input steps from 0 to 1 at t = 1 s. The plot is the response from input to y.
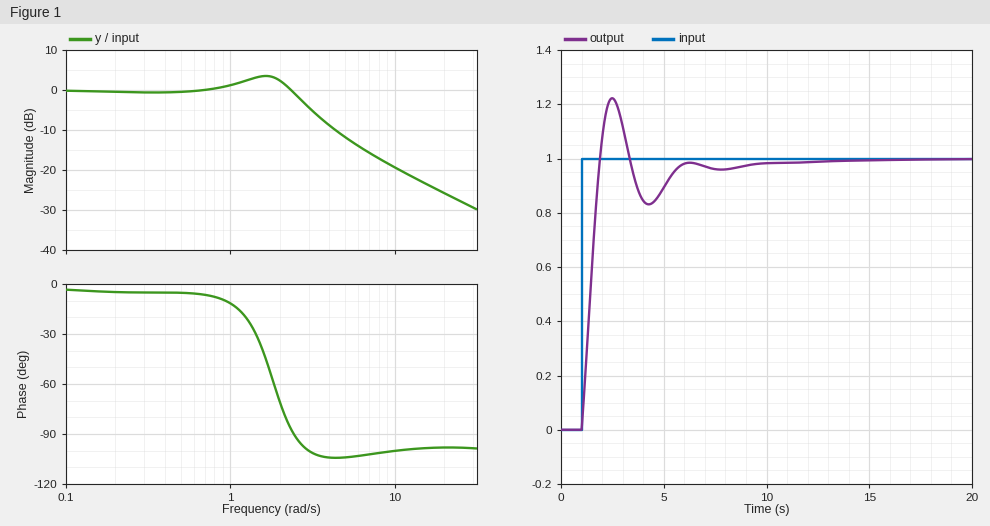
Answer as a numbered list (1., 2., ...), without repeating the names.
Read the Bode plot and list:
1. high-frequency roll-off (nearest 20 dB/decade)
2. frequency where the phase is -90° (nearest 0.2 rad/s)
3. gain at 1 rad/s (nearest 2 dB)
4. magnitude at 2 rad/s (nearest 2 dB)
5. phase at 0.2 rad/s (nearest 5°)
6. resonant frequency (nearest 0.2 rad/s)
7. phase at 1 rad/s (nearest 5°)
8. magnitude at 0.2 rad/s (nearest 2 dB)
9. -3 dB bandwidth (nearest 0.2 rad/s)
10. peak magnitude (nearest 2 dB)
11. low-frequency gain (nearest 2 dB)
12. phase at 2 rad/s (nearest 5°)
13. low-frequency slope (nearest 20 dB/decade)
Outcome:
1. -20 dB/decade
2. 2.4 rad/s
3. 2 dB
4. 2 dB
5. -5°
6. 1.6 rad/s
7. -10°
8. 0 dB
9. 2.8 rad/s
10. 4 dB
11. 0 dB
12. -70°
13. 0 dB/decade
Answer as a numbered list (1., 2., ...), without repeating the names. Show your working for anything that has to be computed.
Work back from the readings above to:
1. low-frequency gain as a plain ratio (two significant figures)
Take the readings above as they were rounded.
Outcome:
1. 10^(0 / 20) = 1.0
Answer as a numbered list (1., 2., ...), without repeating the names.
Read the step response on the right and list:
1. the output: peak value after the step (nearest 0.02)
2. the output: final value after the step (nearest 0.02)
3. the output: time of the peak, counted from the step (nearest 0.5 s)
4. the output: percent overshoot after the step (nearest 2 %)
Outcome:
1. 1.22
2. 1.00
3. 1.5 s
4. 22 %
